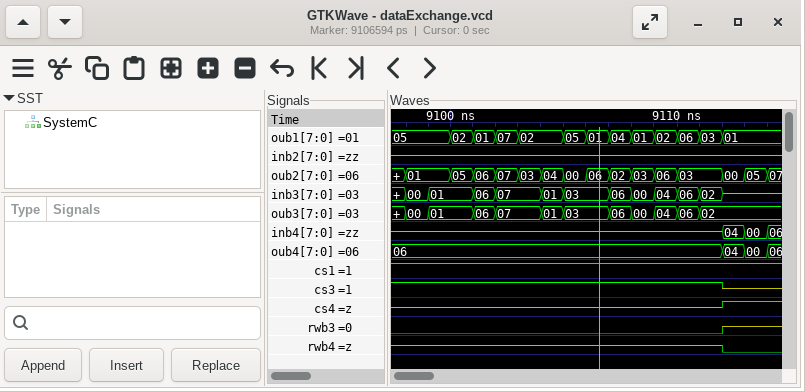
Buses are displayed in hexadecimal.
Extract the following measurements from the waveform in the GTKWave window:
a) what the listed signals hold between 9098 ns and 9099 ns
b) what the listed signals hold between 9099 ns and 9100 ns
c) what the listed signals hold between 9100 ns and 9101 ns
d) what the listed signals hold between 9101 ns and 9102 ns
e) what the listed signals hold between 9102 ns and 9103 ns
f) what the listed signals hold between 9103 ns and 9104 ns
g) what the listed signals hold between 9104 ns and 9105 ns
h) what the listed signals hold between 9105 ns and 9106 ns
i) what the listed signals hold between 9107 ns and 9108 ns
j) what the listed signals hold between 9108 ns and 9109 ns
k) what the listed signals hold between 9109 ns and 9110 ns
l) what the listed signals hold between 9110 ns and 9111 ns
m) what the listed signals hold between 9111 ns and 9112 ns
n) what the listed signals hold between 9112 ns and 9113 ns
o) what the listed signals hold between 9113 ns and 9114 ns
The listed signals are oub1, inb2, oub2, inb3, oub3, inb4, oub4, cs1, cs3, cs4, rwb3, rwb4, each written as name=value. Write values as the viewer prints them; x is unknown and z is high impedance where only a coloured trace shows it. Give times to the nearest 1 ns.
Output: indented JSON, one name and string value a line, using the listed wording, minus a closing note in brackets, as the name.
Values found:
{
  "what the listed signals hold between 9098 ns and 9099 ns": "oub1=05, inb2=z, oub2=01, inb3=00, oub3=00, inb4=z, oub4=06, cs1=1, cs3=1, cs4=z, rwb3=0, rwb4=z",
  "what the listed signals hold between 9099 ns and 9100 ns": "oub1=05, inb2=z, oub2=01, inb3=01, oub3=01, inb4=z, oub4=06, cs1=1, cs3=1, cs4=z, rwb3=0, rwb4=z",
  "what the listed signals hold between 9100 ns and 9101 ns": "oub1=02, inb2=z, oub2=05, inb3=01, oub3=01, inb4=z, oub4=06, cs1=1, cs3=1, cs4=z, rwb3=0, rwb4=z",
  "what the listed signals hold between 9101 ns and 9102 ns": "oub1=01, inb2=z, oub2=06, inb3=06, oub3=06, inb4=z, oub4=06, cs1=1, cs3=1, cs4=z, rwb3=0, rwb4=z",
  "what the listed signals hold between 9102 ns and 9103 ns": "oub1=07, inb2=z, oub2=07, inb3=07, oub3=07, inb4=z, oub4=06, cs1=1, cs3=1, cs4=z, rwb3=0, rwb4=z",
  "what the listed signals hold between 9103 ns and 9104 ns": "oub1=02, inb2=z, oub2=03, inb3=07, oub3=07, inb4=z, oub4=06, cs1=1, cs3=1, cs4=z, rwb3=0, rwb4=z",
  "what the listed signals hold between 9104 ns and 9105 ns": "oub1=02, inb2=z, oub2=04, inb3=01, oub3=01, inb4=z, oub4=06, cs1=1, cs3=1, cs4=z, rwb3=0, rwb4=z",
  "what the listed signals hold between 9105 ns and 9106 ns": "oub1=05, inb2=z, oub2=00, inb3=03, oub3=03, inb4=z, oub4=06, cs1=1, cs3=1, cs4=z, rwb3=0, rwb4=z",
  "what the listed signals hold between 9107 ns and 9108 ns": "oub1=04, inb2=z, oub2=02, inb3=06, oub3=06, inb4=z, oub4=06, cs1=1, cs3=1, cs4=z, rwb3=0, rwb4=z",
  "what the listed signals hold between 9108 ns and 9109 ns": "oub1=01, inb2=z, oub2=03, inb3=00, oub3=00, inb4=z, oub4=06, cs1=1, cs3=1, cs4=z, rwb3=0, rwb4=z",
  "what the listed signals hold between 9109 ns and 9110 ns": "oub1=02, inb2=z, oub2=06, inb3=04, oub3=04, inb4=z, oub4=06, cs1=1, cs3=1, cs4=z, rwb3=0, rwb4=z",
  "what the listed signals hold between 9110 ns and 9111 ns": "oub1=06, inb2=z, oub2=03, inb3=06, oub3=06, inb4=z, oub4=06, cs1=1, cs3=1, cs4=z, rwb3=0, rwb4=z",
  "what the listed signals hold between 9111 ns and 9112 ns": "oub1=03, inb2=z, oub2=03, inb3=02, oub3=02, inb4=z, oub4=06, cs1=1, cs3=1, cs4=z, rwb3=0, rwb4=z",
  "what the listed signals hold between 9112 ns and 9113 ns": "oub1=01, inb2=z, oub2=00, inb3=z, oub3=02, inb4=04, oub4=04, cs1=1, cs3=z, cs4=1, rwb3=z, rwb4=0",
  "what the listed signals hold between 9113 ns and 9114 ns": "oub1=01, inb2=z, oub2=05, inb3=z, oub3=02, inb4=00, oub4=00, cs1=1, cs3=z, cs4=1, rwb3=z, rwb4=0"
}
